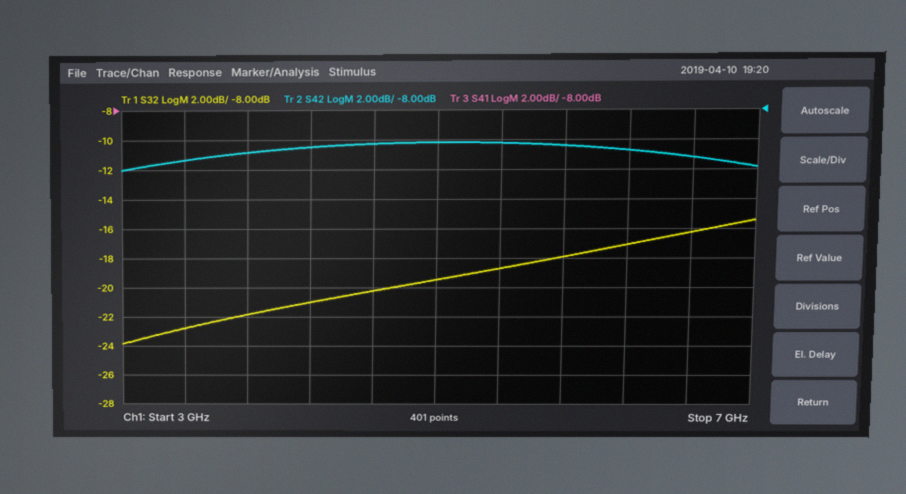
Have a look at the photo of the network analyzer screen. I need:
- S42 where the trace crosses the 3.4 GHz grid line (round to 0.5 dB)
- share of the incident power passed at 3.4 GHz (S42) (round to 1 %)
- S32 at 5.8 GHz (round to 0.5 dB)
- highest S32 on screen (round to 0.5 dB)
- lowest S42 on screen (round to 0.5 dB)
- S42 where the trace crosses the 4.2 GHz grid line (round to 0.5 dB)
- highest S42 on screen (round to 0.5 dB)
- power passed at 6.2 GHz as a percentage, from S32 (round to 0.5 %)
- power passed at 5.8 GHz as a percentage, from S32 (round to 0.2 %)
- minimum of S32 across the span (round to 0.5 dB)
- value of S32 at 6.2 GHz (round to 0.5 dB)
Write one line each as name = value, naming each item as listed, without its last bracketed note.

S42 where the trace crosses the 3.4 GHz grid line = -11.5 dB
share of the incident power passed at 3.4 GHz (S42) = 7 %
S32 at 5.8 GHz = -18.0 dB
highest S32 on screen = -15.5 dB
lowest S42 on screen = -12.0 dB
S42 where the trace crosses the 4.2 GHz grid line = -10.5 dB
highest S42 on screen = -10.0 dB
power passed at 6.2 GHz as a percentage, from S32 = 2.0 %
power passed at 5.8 GHz as a percentage, from S32 = 1.6 %
minimum of S32 across the span = -24.0 dB
value of S32 at 6.2 GHz = -17.0 dB
